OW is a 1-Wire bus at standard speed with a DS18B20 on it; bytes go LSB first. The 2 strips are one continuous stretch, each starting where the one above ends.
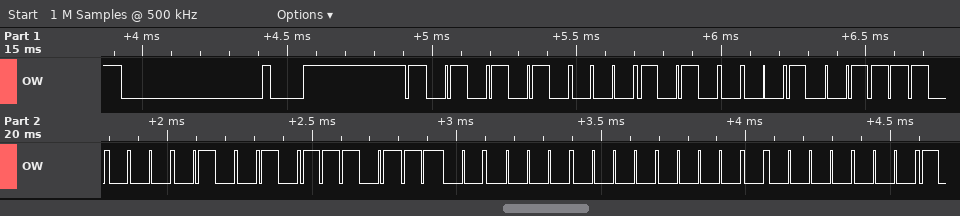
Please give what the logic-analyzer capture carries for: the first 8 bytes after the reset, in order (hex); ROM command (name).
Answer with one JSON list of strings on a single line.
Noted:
["55 28 E4 41 BA 03 00 00", "Match ROM"]
